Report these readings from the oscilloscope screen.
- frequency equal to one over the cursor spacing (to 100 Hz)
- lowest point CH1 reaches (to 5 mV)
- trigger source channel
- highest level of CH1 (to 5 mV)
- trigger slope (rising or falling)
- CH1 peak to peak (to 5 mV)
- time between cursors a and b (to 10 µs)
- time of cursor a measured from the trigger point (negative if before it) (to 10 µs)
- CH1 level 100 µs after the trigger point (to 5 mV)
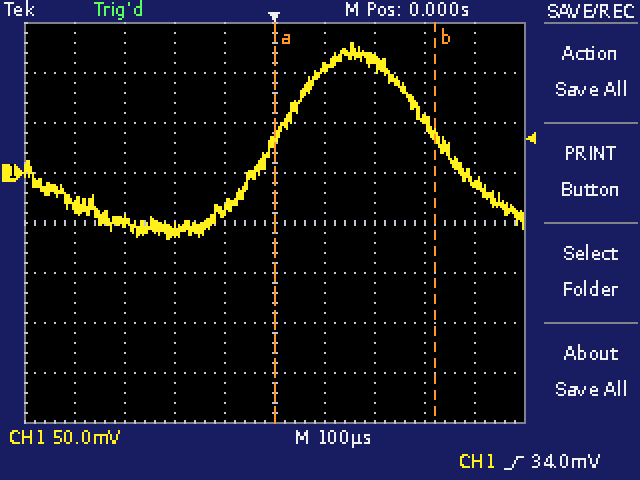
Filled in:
3.1 kHz
-65 mV
CH1
130 mV
rising
195 mV
320 µs
0 µs
105 mV
